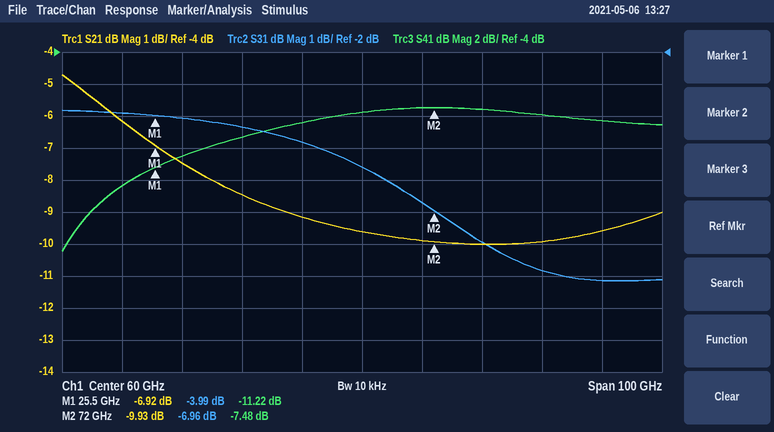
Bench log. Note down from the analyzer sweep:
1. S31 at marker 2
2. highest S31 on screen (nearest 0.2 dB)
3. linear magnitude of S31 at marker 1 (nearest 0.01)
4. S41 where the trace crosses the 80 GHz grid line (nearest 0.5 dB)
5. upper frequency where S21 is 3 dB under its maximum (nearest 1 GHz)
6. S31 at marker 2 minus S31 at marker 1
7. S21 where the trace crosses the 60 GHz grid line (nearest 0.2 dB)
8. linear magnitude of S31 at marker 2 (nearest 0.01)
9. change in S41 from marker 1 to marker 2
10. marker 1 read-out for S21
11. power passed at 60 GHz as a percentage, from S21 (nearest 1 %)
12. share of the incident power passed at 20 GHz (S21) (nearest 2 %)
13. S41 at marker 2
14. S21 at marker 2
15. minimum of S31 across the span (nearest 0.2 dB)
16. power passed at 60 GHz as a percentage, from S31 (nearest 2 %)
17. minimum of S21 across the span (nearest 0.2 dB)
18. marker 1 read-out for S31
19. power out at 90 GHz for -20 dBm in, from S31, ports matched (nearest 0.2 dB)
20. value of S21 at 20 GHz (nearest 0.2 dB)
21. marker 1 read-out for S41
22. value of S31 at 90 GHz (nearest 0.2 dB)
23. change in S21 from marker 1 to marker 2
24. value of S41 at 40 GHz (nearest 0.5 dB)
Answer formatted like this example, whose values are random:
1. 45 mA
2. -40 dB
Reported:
1. -6.96 dB
2. -3.8 dB
3. 0.63
4. -7.5 dB
5. 32 GHz
6. -2.97 dB
7. -9.6 dB
8. 0.45
9. 3.74 dB
10. -6.92 dB
11. 11 %
12. 24 %
13. -7.48 dB
14. -9.93 dB
15. -9.2 dB
16. 28 %
17. -10.0 dB
18. -3.99 dB
19. -28.8 dBm
20. -6.2 dB
21. -11.22 dB
22. -8.8 dB
23. -3.01 dB
24. -9.5 dB
